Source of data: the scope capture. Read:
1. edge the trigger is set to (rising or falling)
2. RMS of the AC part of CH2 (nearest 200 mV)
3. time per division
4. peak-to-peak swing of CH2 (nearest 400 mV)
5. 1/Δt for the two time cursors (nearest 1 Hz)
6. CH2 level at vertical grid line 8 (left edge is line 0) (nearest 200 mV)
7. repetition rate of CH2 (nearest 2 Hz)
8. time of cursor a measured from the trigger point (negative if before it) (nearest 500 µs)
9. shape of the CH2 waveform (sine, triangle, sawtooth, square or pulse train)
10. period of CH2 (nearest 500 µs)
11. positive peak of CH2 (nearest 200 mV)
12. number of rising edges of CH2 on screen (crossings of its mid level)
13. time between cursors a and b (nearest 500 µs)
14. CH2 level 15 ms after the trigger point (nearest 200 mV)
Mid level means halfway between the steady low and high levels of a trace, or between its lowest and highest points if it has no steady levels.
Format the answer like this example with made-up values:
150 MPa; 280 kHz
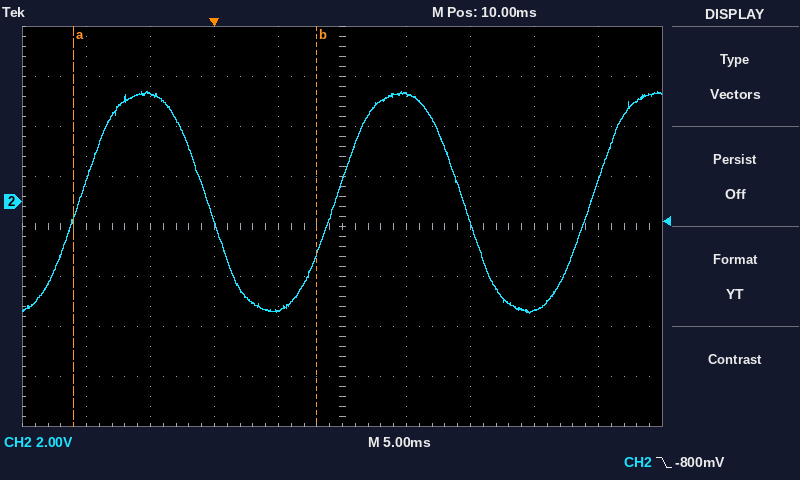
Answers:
falling; 3.2 V; 5 ms; 8.8 V; 53 Hz; -4.4 V; 50 Hz; -11.0 ms; sine; 20.0 ms; 4.4 V; 3; 19.0 ms; 4.2 V
